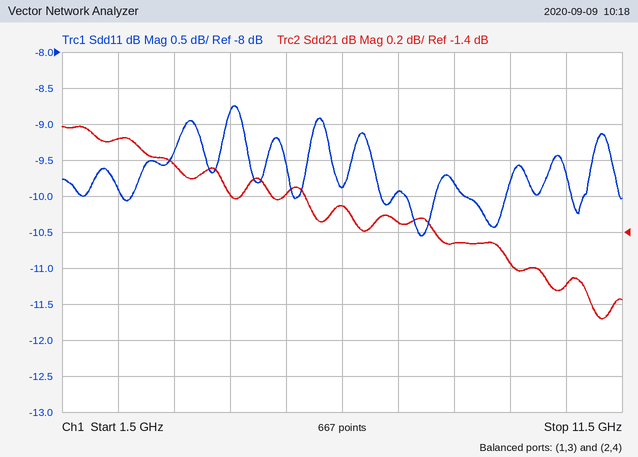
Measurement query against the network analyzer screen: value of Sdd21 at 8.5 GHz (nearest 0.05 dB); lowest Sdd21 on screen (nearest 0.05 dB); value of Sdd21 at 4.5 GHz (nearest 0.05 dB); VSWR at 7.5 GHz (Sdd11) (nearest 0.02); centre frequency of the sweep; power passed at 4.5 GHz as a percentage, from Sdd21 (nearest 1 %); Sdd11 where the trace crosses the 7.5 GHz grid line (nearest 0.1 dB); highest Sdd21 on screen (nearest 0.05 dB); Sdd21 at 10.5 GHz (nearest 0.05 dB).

-1.45 dB
-1.90 dB
-1.20 dB
1.94
6.5 GHz
76 %
-9.9 dB
-0.80 dB
-1.70 dB
